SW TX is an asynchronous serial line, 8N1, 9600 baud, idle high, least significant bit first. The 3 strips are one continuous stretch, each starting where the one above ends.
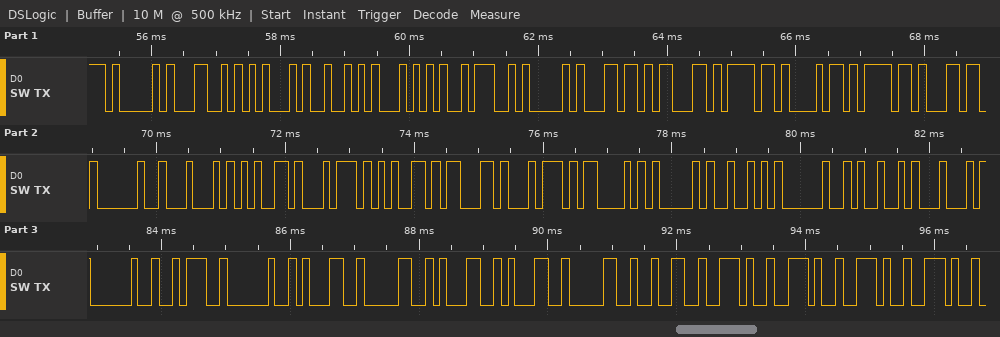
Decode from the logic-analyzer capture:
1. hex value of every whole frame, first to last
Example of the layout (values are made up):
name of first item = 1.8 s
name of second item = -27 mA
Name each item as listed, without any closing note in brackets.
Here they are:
hex value of every whole frame, first to last = 41 4C 45 52 54 3A 41 6C 63 6F 68 6F 6C 20 44 65 74 65 63 74 43 41 52 20 49 44 20 3A 20 31 30 31 31 30 32 2E 2E 2E 2E
